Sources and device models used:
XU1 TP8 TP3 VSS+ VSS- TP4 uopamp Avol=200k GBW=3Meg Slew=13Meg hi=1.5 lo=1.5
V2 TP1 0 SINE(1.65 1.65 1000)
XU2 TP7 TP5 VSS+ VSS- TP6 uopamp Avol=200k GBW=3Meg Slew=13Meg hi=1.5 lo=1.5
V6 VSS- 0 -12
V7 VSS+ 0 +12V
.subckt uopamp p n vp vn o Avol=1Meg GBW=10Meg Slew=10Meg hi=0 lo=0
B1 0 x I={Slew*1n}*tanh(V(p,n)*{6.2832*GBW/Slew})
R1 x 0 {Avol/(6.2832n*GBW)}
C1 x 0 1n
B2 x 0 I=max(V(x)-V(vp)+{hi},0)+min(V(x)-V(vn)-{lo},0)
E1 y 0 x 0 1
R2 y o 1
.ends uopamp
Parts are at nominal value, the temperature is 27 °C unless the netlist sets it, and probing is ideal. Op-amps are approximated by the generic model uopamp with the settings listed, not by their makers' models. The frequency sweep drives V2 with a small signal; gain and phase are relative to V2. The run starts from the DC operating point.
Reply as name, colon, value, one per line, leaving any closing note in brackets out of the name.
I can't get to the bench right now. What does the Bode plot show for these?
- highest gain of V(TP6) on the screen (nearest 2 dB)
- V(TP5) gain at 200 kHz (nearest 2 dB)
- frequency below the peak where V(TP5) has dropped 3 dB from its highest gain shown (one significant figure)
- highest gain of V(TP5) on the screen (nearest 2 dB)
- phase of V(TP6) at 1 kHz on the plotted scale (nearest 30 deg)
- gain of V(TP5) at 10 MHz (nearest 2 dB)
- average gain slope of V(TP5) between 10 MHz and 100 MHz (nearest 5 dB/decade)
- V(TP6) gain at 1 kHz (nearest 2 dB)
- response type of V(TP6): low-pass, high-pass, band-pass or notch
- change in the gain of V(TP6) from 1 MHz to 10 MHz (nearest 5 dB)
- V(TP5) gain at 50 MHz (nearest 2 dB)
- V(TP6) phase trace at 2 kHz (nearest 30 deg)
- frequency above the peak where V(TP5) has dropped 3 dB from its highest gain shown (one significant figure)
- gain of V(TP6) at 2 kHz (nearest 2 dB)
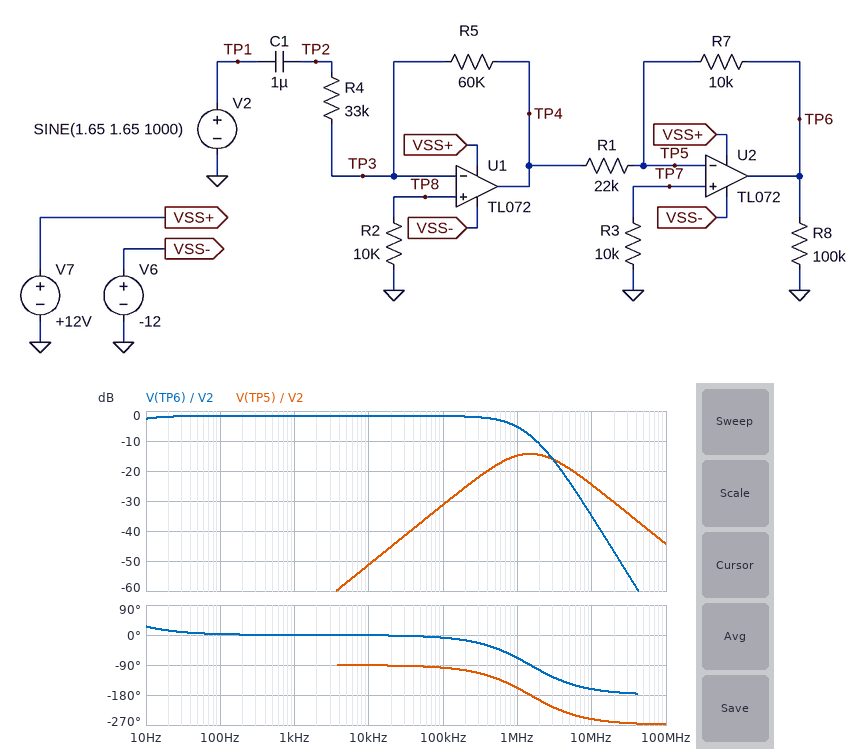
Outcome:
highest gain of V(TP6) on the screen: -2 dB
V(TP5) gain at 200 kHz: -26 dB
frequency below the peak where V(TP5) has dropped 3 dB from its highest gain shown: 600 kHz
highest gain of V(TP5) on the screen: -14 dB
phase of V(TP6) at 1 kHz on the plotted scale: 0 deg
gain of V(TP5) at 10 MHz: -24 dB
average gain slope of V(TP5) between 10 MHz and 100 MHz: -20 dB/decade
V(TP6) gain at 1 kHz: -2 dB
response type of V(TP6): low-pass, high-pass, band-pass or notch: low-pass
change in the gain of V(TP6) from 1 MHz to 10 MHz: -30 dB
V(TP5) gain at 50 MHz: -38 dB
V(TP6) phase trace at 2 kHz: 0 deg
frequency above the peak where V(TP5) has dropped 3 dB from its highest gain shown: 4 MHz
gain of V(TP6) at 2 kHz: -2 dB
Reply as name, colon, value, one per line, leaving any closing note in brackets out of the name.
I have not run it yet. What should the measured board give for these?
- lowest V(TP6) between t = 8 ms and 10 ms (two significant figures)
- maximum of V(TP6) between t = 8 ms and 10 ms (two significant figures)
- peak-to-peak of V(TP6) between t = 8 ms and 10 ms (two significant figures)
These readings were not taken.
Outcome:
lowest V(TP6) between t = 8 ms and 10 ms: -1.4 V
maximum of V(TP6) between t = 8 ms and 10 ms: 1.4 V
peak-to-peak of V(TP6) between t = 8 ms and 10 ms: 2.7 V
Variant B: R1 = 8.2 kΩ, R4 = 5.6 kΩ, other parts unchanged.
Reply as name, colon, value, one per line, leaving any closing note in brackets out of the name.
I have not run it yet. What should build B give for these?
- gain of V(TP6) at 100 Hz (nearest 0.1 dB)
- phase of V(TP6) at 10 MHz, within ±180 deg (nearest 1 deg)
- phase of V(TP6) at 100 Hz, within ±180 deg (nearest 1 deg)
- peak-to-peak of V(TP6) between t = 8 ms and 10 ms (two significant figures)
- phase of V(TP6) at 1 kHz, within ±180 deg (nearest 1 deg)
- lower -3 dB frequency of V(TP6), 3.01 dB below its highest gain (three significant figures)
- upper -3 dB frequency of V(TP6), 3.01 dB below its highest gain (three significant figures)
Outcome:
gain of V(TP6) at 100 Hz: 22.0 dB
phase of V(TP6) at 10 MHz, within ±180 deg: -171 deg
phase of V(TP6) at 100 Hz, within ±180 deg: 16 deg
peak-to-peak of V(TP6) between t = 8 ms and 10 ms: 21 V
phase of V(TP6) at 1 kHz, within ±180 deg: 1 deg
lower -3 dB frequency of V(TP6), 3.01 dB below its highest gain: 28.4 Hz
upper -3 dB frequency of V(TP6), 3.01 dB below its highest gain: 248 kHz
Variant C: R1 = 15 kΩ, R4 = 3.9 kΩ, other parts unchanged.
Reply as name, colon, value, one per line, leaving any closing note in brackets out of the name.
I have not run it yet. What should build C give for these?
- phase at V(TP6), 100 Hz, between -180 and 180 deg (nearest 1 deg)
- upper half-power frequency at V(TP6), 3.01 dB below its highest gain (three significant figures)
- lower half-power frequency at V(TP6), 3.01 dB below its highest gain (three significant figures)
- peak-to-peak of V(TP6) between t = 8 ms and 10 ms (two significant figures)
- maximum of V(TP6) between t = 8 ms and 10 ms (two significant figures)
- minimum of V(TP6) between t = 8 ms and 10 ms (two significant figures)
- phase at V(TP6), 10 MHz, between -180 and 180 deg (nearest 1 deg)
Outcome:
phase at V(TP6), 100 Hz, between -180 and 180 deg: 22 deg
upper half-power frequency at V(TP6), 3.01 dB below its highest gain: 181 kHz
lower half-power frequency at V(TP6), 3.01 dB below its highest gain: 40.8 Hz
peak-to-peak of V(TP6) between t = 8 ms and 10 ms: 14 V
maximum of V(TP6) between t = 8 ms and 10 ms: 7.0 V
minimum of V(TP6) between t = 8 ms and 10 ms: -7.0 V
phase at V(TP6), 10 MHz, between -180 and 180 deg: -169 deg
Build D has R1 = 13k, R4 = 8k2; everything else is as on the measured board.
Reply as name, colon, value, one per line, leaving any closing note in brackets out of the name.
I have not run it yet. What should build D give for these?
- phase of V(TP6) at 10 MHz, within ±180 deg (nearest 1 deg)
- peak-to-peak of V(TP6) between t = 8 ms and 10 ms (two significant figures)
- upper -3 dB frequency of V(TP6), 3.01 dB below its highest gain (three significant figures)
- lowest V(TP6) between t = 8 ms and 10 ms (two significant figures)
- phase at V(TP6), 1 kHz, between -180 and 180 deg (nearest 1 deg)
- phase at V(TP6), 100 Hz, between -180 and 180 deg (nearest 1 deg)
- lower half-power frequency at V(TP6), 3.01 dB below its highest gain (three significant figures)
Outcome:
phase of V(TP6) at 10 MHz, within ±180 deg: -168 deg
peak-to-peak of V(TP6) between t = 8 ms and 10 ms: 16 V
upper -3 dB frequency of V(TP6), 3.01 dB below its highest gain: 346 kHz
lowest V(TP6) between t = 8 ms and 10 ms: -8.1 V
phase at V(TP6), 1 kHz, between -180 and 180 deg: 1 deg
phase at V(TP6), 100 Hz, between -180 and 180 deg: 11 deg
lower half-power frequency at V(TP6), 3.01 dB below its highest gain: 19.4 Hz
